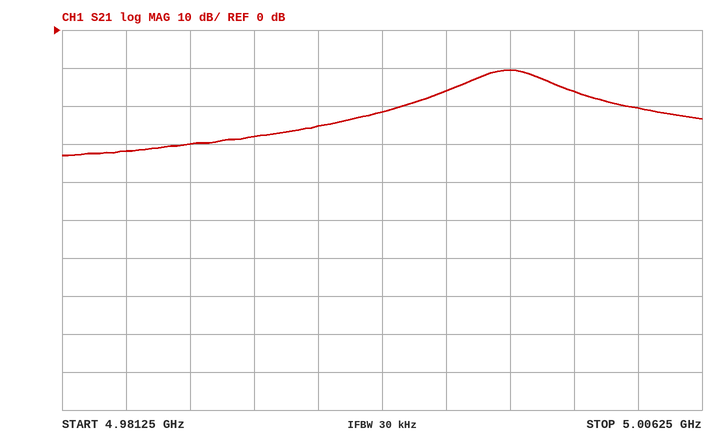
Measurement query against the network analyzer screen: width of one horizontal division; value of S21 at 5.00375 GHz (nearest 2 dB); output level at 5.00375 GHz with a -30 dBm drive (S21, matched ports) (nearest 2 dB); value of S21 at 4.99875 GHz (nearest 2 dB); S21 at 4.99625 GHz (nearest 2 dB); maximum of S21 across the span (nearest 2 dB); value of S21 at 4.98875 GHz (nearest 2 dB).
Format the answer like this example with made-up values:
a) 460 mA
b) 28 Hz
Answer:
a) 2.5 MHz
b) -20 dB
c) -50 dBm
d) -10 dB
e) -16 dB
f) -10 dB
g) -28 dB
